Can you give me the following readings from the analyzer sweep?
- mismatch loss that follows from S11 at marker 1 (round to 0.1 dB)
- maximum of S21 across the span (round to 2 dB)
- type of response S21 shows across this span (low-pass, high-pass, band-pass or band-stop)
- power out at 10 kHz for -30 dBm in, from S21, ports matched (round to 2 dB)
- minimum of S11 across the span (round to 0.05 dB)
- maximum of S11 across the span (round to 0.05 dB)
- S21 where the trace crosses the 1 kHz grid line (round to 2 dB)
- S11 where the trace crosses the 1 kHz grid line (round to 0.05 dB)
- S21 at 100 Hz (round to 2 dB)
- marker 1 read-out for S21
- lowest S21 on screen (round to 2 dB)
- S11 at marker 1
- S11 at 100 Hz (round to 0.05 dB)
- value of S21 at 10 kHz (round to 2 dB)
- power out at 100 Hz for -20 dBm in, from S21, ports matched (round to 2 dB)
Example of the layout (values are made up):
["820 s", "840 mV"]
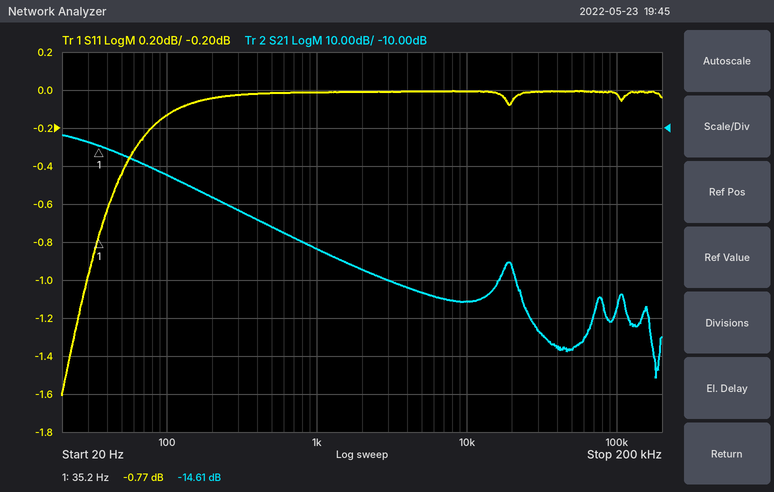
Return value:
["7.9 dB", "-12 dB", "low-pass", "-86 dBm", "-1.60 dB", "0.00 dB", "-42 dB", "0.00 dB", "-22 dB", "-14.61 dB", "-76 dB", "-0.77 dB", "-0.15 dB", "-56 dB", "-42 dBm"]
